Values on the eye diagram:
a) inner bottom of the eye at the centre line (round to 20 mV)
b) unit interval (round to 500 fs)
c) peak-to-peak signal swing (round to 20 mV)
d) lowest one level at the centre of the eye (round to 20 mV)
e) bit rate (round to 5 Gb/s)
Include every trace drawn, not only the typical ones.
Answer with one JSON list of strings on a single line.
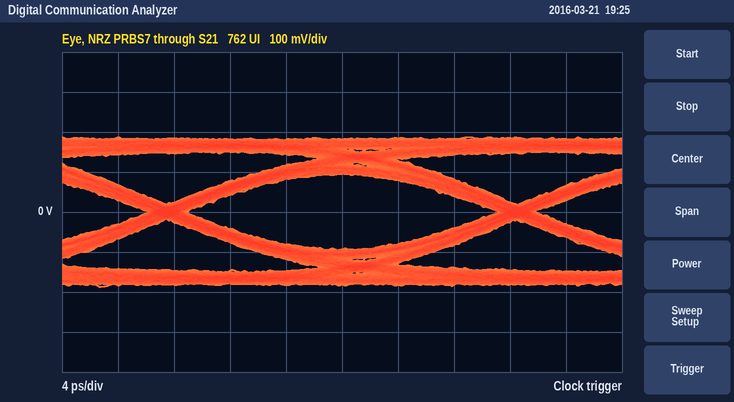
["-100 mV", "25.0 ps", "380 mV", "100 mV", "40 Gb/s"]
